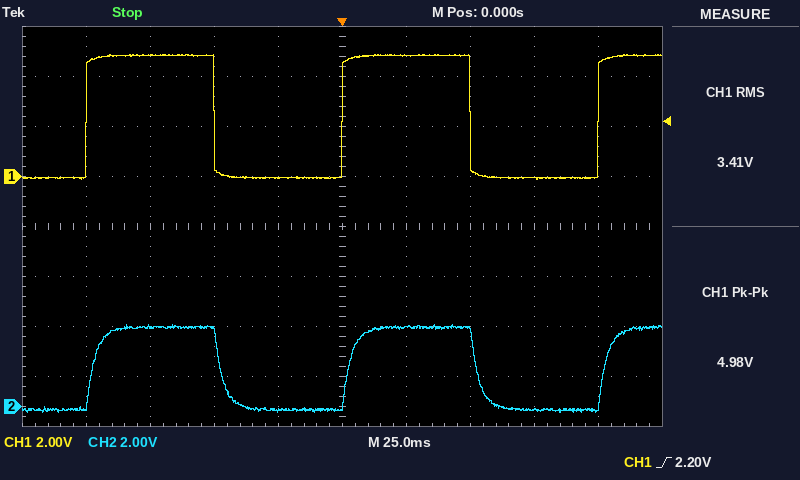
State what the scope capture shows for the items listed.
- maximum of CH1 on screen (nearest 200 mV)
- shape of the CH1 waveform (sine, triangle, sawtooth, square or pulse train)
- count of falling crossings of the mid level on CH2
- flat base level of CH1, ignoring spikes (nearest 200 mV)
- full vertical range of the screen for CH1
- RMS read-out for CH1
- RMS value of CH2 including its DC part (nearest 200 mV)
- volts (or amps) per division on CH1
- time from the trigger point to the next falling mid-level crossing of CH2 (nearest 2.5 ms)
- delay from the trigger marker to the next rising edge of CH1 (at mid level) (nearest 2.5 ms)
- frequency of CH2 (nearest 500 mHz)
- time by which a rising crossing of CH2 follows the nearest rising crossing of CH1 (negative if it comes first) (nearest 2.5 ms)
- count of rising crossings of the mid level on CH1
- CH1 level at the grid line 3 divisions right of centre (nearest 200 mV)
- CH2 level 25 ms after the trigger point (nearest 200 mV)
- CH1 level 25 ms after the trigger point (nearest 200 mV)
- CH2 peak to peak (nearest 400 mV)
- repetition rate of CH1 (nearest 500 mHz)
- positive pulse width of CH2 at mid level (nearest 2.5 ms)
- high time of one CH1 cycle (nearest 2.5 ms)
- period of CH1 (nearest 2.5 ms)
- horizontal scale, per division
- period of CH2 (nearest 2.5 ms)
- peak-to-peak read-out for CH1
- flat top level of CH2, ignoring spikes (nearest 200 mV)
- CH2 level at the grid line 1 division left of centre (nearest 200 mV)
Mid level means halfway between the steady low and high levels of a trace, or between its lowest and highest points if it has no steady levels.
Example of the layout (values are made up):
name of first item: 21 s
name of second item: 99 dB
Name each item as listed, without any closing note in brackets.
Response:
maximum of CH1 on screen: 4.8 V
shape of the CH1 waveform: square
count of falling crossings of the mid level on CH2: 2
flat base level of CH1, ignoring spikes: 0.0 V
full vertical range of the screen for CH1: 16 V
RMS read-out for CH1: 3.41 V
RMS value of CH2 including its DC part: 2.2 V
volts (or amps) per division on CH1: 2 V
time from the trigger point to the next falling mid-level crossing of CH2: 52.5 ms
delay from the trigger marker to the next rising edge of CH1 (at mid level): 100.0 ms
frequency of CH2: 10.0 Hz
time by which a rising crossing of CH2 follows the nearest rising crossing of CH1 (negative if it comes first): +2.5 ms
count of rising crossings of the mid level on CH1: 3
CH1 level at the grid line 3 divisions right of centre: 0.0 V
CH2 level 25 ms after the trigger point: 3.2 V
CH1 level 25 ms after the trigger point: 4.8 V
CH2 peak to peak: 3.6 V
repetition rate of CH1: 10.0 Hz
positive pulse width of CH2 at mid level: 50.0 ms
high time of one CH1 cycle: 50.0 ms
period of CH1: 100.0 ms
horizontal scale, per division: 25 ms
period of CH2: 100.0 ms
peak-to-peak read-out for CH1: 4.98 V
flat top level of CH2, ignoring spikes: 3.2 V
CH2 level at the grid line 1 division left of centre: -200 mV
